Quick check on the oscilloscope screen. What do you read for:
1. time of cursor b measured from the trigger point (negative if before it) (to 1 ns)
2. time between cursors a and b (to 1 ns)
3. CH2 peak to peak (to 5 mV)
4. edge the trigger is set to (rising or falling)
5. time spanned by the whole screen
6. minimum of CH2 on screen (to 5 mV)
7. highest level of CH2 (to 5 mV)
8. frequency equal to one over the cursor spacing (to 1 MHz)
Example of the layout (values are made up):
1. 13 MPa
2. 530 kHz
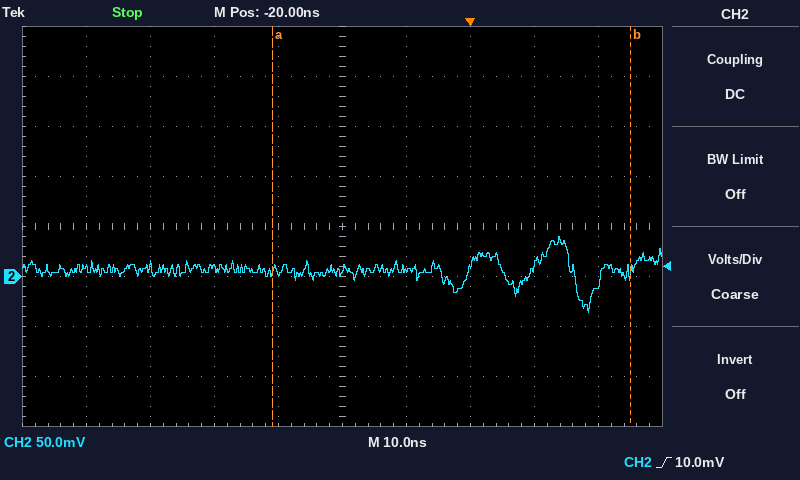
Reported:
1. +25 ns
2. 56 ns
3. 75 mV
4. rising
5. 100 ns
6. -35 mV
7. 40 mV
8. 18 MHz
